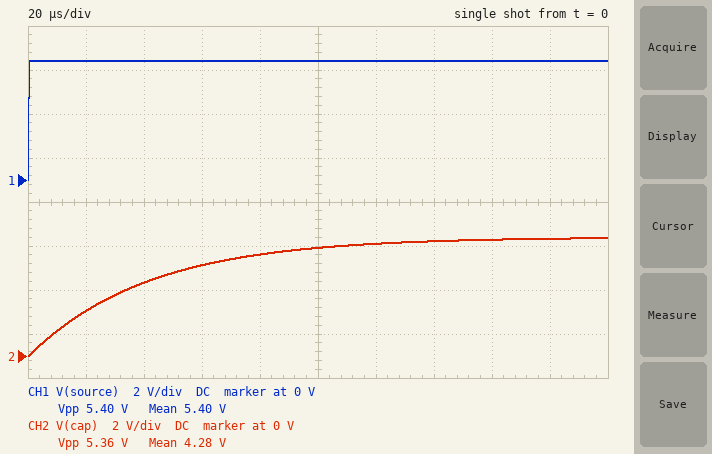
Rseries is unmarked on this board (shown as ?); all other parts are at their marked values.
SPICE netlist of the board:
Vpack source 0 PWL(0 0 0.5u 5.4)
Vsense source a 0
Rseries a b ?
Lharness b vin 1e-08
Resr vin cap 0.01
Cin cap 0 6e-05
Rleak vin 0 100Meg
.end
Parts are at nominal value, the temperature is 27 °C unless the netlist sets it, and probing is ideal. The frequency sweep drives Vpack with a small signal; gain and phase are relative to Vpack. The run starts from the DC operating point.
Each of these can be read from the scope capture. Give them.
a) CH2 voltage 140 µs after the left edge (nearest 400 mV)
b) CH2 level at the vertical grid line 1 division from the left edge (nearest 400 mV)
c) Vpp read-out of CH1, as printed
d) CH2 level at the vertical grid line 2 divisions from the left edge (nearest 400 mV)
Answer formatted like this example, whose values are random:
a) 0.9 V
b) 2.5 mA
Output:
a) 5.2 V
b) 2.0 V
c) 5.40 V
d) 3.2 V
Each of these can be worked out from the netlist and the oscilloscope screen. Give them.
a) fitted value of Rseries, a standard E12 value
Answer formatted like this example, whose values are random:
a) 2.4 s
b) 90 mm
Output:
a) 0.68 Ω
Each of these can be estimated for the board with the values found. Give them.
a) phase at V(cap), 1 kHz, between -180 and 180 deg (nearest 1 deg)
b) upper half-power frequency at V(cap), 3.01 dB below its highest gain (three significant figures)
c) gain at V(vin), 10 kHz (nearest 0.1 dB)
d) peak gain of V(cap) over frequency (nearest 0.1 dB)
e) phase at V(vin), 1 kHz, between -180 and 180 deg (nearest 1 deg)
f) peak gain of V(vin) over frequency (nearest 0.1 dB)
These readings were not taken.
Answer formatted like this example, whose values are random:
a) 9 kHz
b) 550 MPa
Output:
a) -15 deg
b) 3.85 kHz
c) -8.9 dB
d) 0 dB
e) -14 deg
f) 0 dB
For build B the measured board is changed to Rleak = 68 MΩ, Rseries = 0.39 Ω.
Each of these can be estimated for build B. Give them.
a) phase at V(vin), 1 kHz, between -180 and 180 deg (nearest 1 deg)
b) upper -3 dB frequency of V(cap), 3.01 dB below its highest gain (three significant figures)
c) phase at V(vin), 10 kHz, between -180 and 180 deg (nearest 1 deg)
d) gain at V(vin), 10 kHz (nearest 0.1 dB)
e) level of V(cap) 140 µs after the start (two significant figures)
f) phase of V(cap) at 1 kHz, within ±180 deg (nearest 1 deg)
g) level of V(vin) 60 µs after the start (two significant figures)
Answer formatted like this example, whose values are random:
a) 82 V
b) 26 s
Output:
a) -8 deg
b) 6.64 kHz
c) -54 deg
d) -5.1 dB
e) 5.4 V
f) -9 deg
g) 5.0 V
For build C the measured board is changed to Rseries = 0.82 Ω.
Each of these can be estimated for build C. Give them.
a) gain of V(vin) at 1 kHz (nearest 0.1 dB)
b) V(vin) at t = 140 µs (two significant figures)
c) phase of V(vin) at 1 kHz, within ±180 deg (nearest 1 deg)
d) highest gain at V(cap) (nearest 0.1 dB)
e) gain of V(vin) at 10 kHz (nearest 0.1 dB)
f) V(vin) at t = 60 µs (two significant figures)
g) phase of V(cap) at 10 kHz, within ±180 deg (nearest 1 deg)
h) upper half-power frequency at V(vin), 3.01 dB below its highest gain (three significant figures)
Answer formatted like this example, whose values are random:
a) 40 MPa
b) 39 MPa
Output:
a) -0.4 dB
b) 5.1 V
c) -17 deg
d) 0 dB
e) -10.3 dB
f) 3.8 V
g) -72 deg
h) 3.20 kHz
